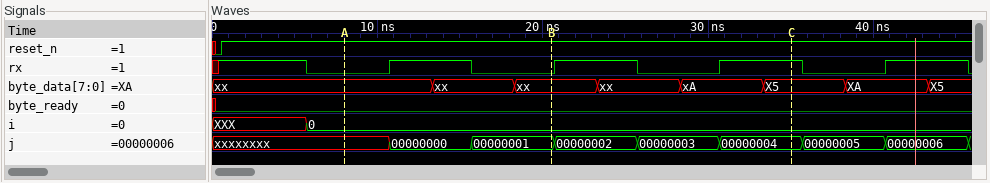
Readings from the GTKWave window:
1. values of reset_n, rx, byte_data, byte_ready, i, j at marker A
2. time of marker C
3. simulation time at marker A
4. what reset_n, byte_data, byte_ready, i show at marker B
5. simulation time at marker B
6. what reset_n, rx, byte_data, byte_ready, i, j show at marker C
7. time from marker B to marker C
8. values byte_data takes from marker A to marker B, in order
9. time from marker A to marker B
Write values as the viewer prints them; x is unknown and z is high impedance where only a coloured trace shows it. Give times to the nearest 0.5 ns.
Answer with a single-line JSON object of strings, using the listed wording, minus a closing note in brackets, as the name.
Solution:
{"values of reset_n, rx, byte_data, byte_ready, i, j at marker A": "reset_n=1, rx=0, byte_data=xx, byte_ready=0, i=0, j=xxxxxxxx", "time of marker C": "35 ns", "simulation time at marker A": "8 ns", "what reset_n, byte_data, byte_ready, i show at marker B": "reset_n=1, byte_data=xx, byte_ready=0, i=0", "simulation time at marker B": "20.5 ns", "what reset_n, rx, byte_data, byte_ready, i, j show at marker C": "reset_n=1, rx=1, byte_data=X5, byte_ready=0, i=0, j=00000004", "time from marker B to marker C": "14.5 ns", "values byte_data takes from marker A to marker B, in order": "xx, xx, xx", "time from marker A to marker B": "12.5 ns"}
